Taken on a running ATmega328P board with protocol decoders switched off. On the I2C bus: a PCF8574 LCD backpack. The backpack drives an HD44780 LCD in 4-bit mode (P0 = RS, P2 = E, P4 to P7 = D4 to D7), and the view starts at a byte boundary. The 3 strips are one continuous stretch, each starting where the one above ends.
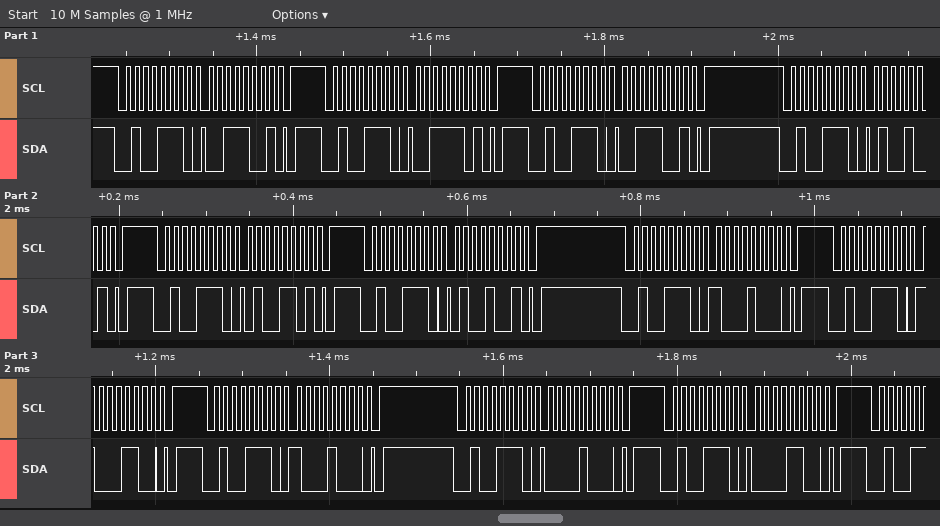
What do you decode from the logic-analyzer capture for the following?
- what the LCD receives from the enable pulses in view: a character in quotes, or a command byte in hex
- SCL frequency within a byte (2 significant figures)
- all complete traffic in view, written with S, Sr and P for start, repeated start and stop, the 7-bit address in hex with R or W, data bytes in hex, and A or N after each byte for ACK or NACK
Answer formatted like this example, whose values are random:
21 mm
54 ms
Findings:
'4'
100 kHz
S 27W A 39 A P S 27W A 3D A P S 27W A 39 A P S 27W A 49 A P S 27W A 4D A P S 27W A 49 A P S 27W A 88 A P S 27W A 8C A P S 27W A 88 A P S 27W A 08 A P S 27W A 0C A P
